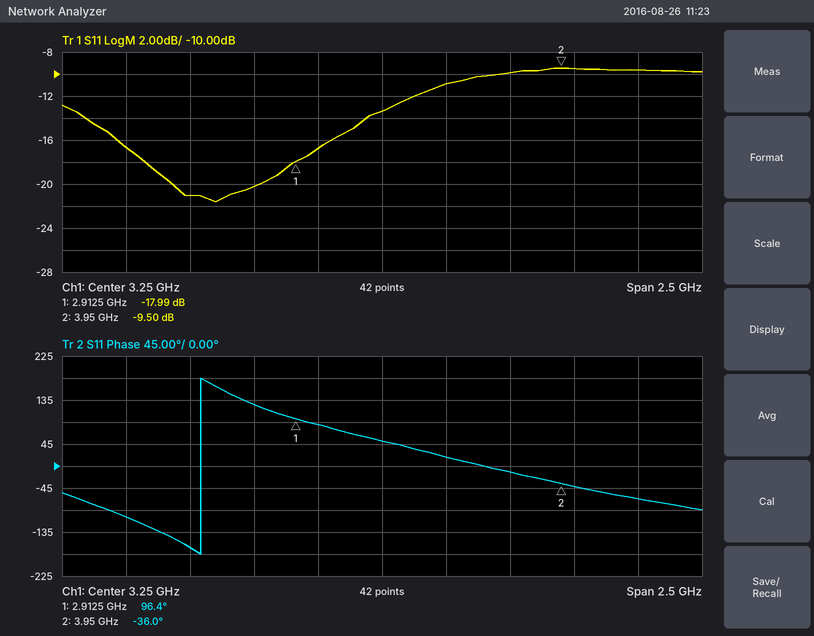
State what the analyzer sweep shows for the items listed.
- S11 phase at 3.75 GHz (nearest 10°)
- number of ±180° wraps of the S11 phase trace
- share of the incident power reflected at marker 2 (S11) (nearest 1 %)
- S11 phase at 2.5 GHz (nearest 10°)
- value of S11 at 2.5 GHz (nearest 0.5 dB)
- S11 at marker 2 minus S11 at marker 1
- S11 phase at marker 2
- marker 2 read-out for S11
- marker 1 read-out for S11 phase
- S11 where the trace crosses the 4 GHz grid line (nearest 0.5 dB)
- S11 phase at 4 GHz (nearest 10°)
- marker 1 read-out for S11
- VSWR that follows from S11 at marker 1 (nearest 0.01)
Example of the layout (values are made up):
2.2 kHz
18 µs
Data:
-10°
1
11 %
-170°
-21.0 dB
8.49 dB
-36.0°
-9.50 dB
96.4°
-9.5 dB
-40°
-17.99 dB
1.29
